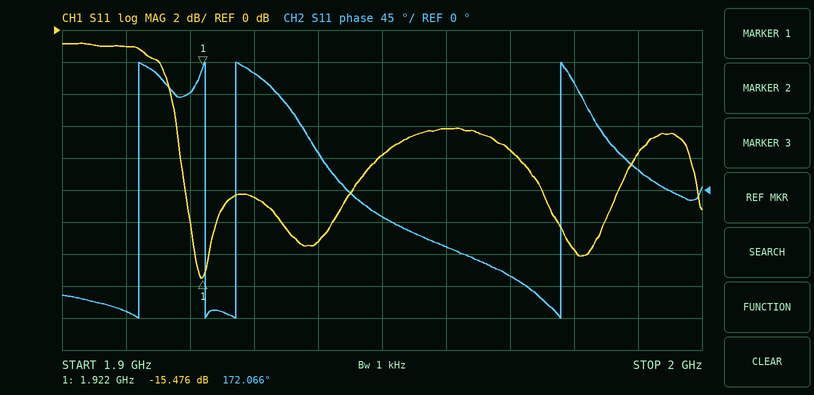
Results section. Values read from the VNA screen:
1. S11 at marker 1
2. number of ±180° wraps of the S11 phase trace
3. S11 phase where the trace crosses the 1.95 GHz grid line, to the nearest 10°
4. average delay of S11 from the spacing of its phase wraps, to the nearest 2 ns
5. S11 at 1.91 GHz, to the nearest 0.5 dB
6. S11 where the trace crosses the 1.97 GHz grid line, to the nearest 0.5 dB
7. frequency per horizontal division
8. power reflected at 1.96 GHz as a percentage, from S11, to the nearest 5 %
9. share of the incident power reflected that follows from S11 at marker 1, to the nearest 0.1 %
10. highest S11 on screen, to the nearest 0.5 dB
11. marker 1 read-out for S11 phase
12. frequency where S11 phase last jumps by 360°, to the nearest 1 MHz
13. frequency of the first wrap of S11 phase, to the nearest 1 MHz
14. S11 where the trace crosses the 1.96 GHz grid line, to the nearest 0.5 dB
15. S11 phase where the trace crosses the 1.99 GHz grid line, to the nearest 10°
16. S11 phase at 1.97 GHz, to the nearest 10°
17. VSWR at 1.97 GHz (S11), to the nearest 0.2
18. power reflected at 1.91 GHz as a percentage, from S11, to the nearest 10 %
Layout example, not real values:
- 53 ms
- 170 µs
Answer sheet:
- -15.476 dB
- 4
- -40°
- 46 ns
- -1.0 dB
- -7.5 dB
- 10 MHz
- 25 %
- 2.8 %
- -1.0 dB
- 172.066°
- 1.978 GHz
- 1.912 GHz
- -6.0 dB
- 30°
- -120°
- 2.4
- 80 %
